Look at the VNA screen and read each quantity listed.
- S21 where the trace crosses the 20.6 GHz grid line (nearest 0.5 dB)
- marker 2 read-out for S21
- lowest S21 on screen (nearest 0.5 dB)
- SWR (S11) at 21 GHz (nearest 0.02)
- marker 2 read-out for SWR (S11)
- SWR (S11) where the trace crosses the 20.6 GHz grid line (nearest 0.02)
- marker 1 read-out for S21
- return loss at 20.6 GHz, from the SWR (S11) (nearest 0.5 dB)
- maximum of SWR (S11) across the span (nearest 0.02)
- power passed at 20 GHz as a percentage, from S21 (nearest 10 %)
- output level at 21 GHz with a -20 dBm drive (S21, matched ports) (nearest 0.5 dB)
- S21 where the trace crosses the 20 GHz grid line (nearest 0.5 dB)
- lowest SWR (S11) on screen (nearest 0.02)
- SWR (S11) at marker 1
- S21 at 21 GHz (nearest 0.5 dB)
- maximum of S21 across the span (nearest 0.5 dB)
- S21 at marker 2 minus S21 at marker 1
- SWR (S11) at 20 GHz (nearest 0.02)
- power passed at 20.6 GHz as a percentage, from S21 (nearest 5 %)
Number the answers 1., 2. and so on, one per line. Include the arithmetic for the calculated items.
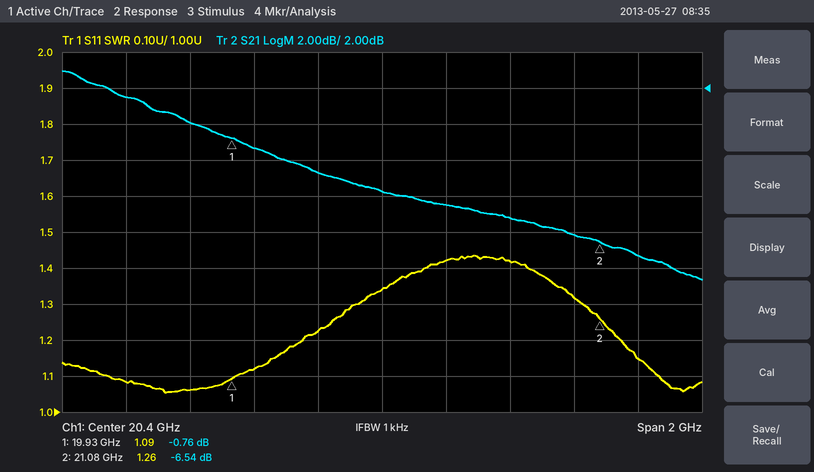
1. -4.5 dB
2. -6.54 dB
3. -8.5 dB
4. 1.32
5. 1.26
6. 1.42
7. -0.76 dB
8. −20 log10((1.42 − 1)/(1.42 + 1)) ≈ 15.2 dB, so 15.0 dB to the nearest 0.5 dB
9. 1.44
10. 10^(-1.5/10) ≈ 70.8 %, so 70 % to the nearest 10 %
11. -20 dBm + (-6.0 dB) = -26.0 dBm
12. -1.5 dB
13. 1.06
14. 1.09
15. -6.0 dB
16. 3.0 dB
17. -6.54 − (-0.76) = -5.78 dB
18. 1.12
19. 10^(-4.5/10) ≈ 35 %
